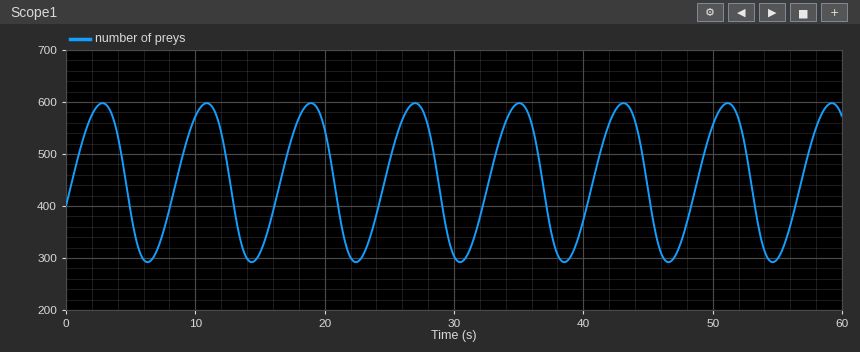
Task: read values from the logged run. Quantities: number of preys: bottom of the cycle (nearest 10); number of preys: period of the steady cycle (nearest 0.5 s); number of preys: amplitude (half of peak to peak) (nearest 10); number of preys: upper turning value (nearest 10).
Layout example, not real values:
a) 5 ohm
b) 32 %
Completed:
a) 290
b) 8.0 s
c) 150
d) 600
